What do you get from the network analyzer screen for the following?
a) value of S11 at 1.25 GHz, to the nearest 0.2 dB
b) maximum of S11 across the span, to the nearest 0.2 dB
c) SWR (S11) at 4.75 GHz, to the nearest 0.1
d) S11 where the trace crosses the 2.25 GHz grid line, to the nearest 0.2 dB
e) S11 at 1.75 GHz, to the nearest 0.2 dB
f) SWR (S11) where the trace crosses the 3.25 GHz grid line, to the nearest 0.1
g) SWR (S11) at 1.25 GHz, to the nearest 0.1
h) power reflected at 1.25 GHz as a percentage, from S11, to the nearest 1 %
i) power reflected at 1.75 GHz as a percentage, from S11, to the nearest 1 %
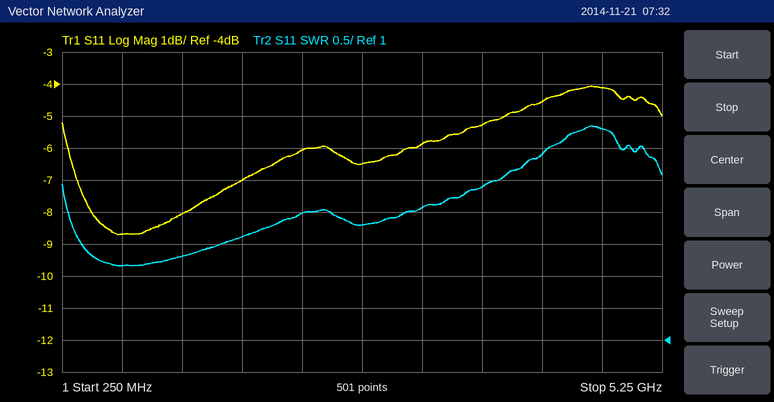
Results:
-8.0 dB
-4.0 dB
4.3
-6.0 dB
-7.0 dB
3.1
2.3
16 %
20 %
